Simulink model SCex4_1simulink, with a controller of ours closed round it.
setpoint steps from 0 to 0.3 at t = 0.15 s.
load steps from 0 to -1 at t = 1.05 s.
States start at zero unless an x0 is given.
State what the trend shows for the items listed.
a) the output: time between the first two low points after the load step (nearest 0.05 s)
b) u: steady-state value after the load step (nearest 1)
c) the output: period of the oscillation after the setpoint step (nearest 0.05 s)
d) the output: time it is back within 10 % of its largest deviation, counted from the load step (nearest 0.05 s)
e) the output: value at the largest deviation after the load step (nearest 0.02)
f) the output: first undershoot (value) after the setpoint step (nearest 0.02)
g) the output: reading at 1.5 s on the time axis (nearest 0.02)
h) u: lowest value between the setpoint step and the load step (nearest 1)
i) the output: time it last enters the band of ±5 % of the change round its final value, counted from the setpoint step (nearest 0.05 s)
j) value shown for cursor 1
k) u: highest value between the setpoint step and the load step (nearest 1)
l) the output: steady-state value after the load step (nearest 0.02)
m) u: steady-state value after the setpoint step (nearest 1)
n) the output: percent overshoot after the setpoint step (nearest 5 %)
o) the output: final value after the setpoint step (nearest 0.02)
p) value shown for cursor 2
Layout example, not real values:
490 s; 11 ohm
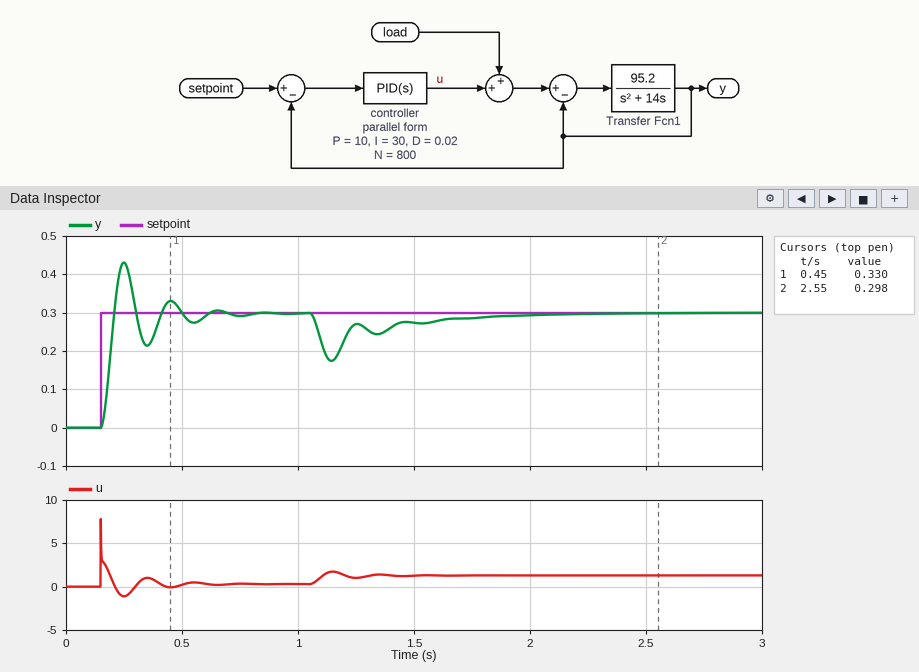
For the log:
0.20 s; 1; 0.20 s; 0.75 s; 0.18; 0.22; 0.28; -1; 0.45 s; 0.330; 8; 0.30; 0; 45 %; 0.30; 0.298
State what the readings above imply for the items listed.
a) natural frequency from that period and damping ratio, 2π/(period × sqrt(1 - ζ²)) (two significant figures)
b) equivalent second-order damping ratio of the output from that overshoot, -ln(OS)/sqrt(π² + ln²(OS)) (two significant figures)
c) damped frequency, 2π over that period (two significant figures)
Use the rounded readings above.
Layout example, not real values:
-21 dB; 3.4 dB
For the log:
32 rad/s; 0.25; 31 rad/s
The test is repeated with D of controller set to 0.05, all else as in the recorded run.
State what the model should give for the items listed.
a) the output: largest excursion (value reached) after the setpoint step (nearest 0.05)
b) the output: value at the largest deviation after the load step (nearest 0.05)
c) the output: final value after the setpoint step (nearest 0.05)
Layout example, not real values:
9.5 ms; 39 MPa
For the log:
0.40; 0.20; 0.30
